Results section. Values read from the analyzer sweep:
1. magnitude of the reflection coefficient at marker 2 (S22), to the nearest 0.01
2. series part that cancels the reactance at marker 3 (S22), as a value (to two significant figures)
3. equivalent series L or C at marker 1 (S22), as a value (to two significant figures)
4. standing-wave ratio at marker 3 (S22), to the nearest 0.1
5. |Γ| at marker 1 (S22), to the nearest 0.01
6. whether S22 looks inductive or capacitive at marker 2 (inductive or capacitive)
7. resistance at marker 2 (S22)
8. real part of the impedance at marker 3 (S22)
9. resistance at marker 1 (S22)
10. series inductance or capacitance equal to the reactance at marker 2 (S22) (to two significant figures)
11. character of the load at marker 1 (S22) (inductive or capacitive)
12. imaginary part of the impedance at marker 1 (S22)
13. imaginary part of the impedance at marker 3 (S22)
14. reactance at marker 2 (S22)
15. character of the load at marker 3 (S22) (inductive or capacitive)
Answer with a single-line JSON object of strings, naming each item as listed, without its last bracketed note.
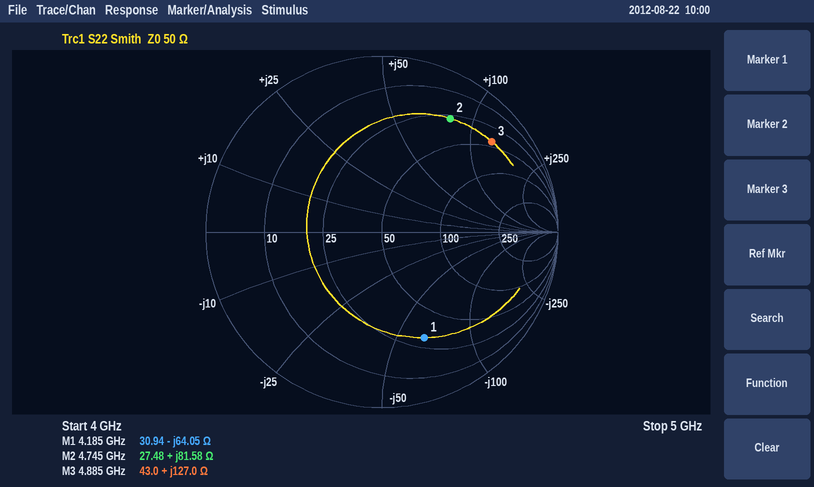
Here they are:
{"magnitude of the reflection coefficient at marker 2 (S22), to the nearest 0.01": "0.75", "series part that cancels the reactance at marker 3 (S22), as a value": "260 fF", "equivalent series L or C at marker 1 (S22), as a value": "590 fF", "standing-wave ratio at marker 3 (S22), to the nearest 0.1": "9.4", "|Γ| at marker 1 (S22), to the nearest 0.01": "0.65", "whether S22 looks inductive or capacitive at marker 2": "inductive", "resistance at marker 2": "27.48 Ω", "real part of the impedance at marker 3": "43.0 Ω", "resistance at marker 1": "30.94 Ω", "series inductance or capacitance equal to the reactance at marker 2 (S22)": "2.7 nH", "character of the load at marker 1 (S22)": "capacitive", "imaginary part of the impedance at marker 1": "-64.05 Ω", "imaginary part of the impedance at marker 3": "+127.0 Ω", "reactance at marker 2": "+81.58 Ω", "character of the load at marker 3 (S22)": "inductive"}
